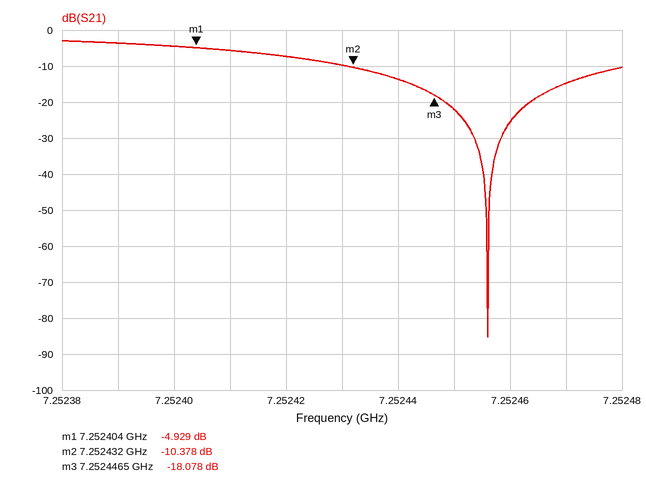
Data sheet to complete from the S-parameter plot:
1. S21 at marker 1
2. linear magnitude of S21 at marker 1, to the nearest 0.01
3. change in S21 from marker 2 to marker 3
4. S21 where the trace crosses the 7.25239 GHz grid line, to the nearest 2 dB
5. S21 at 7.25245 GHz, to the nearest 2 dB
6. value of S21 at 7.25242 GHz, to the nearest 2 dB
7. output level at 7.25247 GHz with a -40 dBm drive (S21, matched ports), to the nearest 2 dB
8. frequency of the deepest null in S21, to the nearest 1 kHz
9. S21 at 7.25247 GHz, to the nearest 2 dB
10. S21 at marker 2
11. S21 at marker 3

-4.929 dB
0.57
-7.700 dB
-4 dB
-22 dB
-8 dB
-54 dBm
7.252456 GHz
-14 dB
-10.378 dB
-18.078 dB
